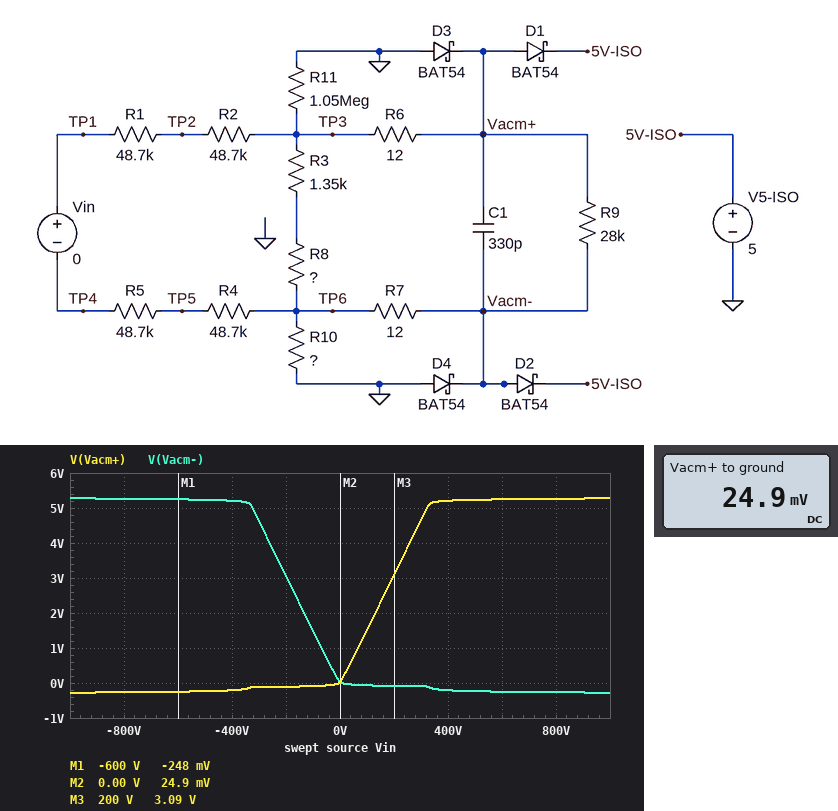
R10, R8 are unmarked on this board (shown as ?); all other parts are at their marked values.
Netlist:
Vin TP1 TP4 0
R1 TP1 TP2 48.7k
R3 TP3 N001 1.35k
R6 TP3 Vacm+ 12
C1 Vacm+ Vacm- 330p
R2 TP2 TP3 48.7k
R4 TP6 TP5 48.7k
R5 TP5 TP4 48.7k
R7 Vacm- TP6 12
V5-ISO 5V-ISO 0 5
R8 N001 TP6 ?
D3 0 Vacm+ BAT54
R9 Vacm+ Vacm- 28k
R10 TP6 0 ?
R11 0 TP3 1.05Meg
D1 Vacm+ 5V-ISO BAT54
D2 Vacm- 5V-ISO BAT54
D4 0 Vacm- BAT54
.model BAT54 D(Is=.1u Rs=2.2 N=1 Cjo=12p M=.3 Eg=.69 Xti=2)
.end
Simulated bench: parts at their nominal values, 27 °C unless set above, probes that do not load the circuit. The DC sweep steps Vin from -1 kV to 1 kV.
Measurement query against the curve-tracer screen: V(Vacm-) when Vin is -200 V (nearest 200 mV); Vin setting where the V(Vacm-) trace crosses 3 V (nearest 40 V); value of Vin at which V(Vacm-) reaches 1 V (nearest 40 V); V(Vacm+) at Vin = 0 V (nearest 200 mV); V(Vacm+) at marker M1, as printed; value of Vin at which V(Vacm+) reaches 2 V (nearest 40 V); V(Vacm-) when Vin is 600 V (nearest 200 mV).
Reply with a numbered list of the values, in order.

1. 3.0 V
2. -200 V
3. -80 V
4. 0 V
5. -248 mV
6. 120 V
7. -200 mV
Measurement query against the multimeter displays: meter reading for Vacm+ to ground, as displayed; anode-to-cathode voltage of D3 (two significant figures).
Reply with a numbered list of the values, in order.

1. 24.9 mV
2. -25 mV
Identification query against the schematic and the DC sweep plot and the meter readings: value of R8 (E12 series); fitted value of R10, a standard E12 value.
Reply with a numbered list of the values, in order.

1. 2.2 kΩ
2. 470 kΩ
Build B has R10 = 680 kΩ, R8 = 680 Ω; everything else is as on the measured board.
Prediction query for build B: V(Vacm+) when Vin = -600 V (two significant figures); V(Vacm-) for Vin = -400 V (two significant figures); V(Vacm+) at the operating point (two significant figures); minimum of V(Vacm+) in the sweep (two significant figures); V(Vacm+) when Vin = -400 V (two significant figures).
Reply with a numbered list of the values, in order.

1. -200 mV
2. 3.7 V
3. 28 mV
4. -260 mV
5. -100 mV
